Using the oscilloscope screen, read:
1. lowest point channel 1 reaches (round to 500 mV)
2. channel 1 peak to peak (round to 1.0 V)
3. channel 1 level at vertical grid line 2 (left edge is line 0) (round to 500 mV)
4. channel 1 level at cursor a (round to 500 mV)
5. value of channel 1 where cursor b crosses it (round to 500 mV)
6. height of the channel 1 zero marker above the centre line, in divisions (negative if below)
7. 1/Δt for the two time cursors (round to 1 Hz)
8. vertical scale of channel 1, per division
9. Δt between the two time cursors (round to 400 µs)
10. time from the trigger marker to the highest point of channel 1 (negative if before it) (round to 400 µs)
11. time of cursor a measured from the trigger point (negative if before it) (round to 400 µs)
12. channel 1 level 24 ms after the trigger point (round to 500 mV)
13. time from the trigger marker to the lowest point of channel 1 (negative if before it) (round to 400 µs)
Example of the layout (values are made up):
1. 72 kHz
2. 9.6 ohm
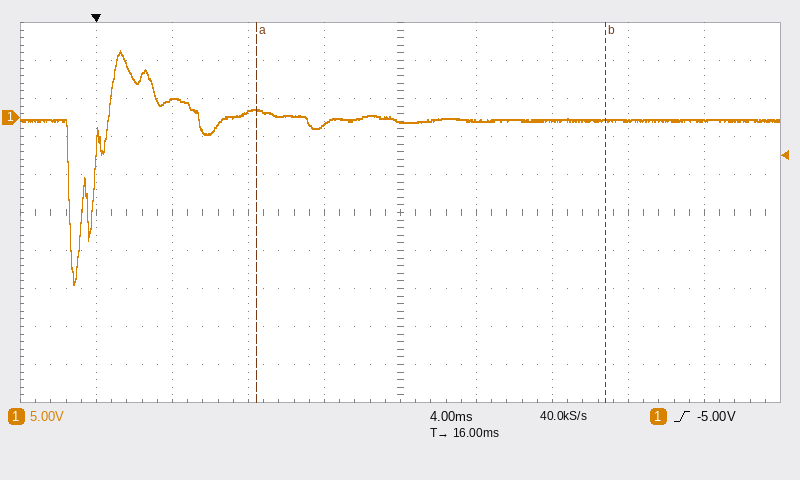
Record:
1. -22.0 V
2. 31.0 V
3. 2.5 V
4. 1.0 V
5. -500 mV
6. +2.5 div
7. 54 Hz
8. 5 V
9. 18.4 ms
10. +1.2 ms
11. +8.4 ms
12. -500 mV
13. -1.2 ms
